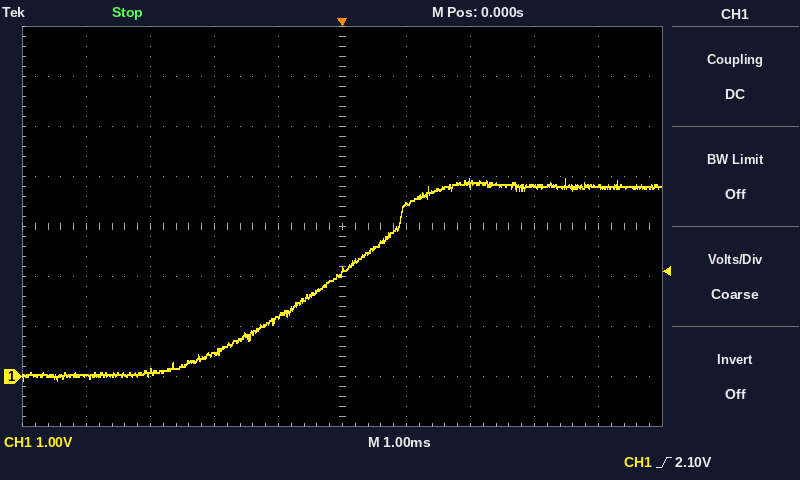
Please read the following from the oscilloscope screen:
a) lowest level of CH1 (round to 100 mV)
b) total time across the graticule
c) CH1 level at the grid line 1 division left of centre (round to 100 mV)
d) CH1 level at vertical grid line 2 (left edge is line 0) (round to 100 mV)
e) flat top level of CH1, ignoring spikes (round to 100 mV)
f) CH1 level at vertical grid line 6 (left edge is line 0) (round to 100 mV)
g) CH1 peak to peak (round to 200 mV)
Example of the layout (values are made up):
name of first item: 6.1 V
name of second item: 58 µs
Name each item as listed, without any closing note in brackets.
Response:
lowest level of CH1: -100 mV
total time across the graticule: 10 ms
CH1 level at the grid line 1 division left of centre: 1.2 V
CH1 level at vertical grid line 2 (left edge is line 0): 100 mV
flat top level of CH1, ignoring spikes: 3.8 V
CH1 level at vertical grid line 6 (left edge is line 0): 3.4 V
CH1 peak to peak: 4.0 V
